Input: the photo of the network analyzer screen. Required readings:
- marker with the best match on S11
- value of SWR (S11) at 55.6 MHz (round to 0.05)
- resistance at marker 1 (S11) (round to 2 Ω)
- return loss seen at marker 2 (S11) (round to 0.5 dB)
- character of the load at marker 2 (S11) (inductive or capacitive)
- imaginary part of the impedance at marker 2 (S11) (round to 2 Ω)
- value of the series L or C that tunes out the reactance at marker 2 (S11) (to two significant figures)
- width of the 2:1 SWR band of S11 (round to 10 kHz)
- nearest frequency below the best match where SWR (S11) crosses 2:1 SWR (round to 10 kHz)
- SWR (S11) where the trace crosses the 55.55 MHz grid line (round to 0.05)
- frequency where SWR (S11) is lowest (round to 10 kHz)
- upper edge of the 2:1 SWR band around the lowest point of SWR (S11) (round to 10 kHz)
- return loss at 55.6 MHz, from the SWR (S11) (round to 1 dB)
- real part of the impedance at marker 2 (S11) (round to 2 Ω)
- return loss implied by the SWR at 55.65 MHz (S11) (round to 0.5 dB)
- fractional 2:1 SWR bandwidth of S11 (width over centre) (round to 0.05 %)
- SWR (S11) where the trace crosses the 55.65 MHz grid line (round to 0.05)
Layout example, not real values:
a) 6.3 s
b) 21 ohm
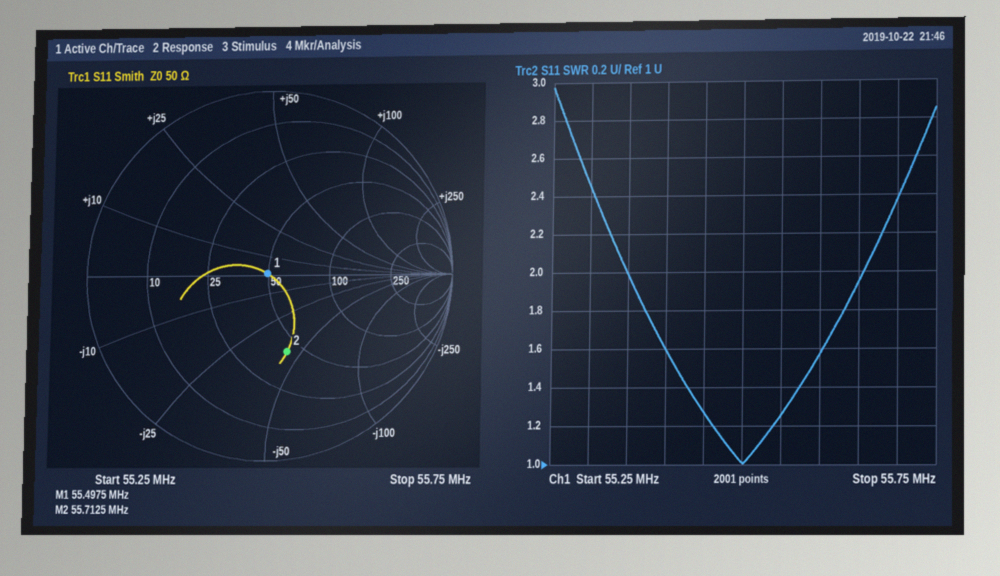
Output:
a) marker 1
b) 1.55
c) 50 Ω
d) 7.5 dB
e) capacitive
f) -42 Ω
g) 120 nH
h) 310 kHz
i) 55.35 MHz
j) 1.25
k) 55.50 MHz
l) 55.66 MHz
m) 13 dB
n) 42 Ω
o) 10.0 dB
p) 0.55 %
q) 1.95
